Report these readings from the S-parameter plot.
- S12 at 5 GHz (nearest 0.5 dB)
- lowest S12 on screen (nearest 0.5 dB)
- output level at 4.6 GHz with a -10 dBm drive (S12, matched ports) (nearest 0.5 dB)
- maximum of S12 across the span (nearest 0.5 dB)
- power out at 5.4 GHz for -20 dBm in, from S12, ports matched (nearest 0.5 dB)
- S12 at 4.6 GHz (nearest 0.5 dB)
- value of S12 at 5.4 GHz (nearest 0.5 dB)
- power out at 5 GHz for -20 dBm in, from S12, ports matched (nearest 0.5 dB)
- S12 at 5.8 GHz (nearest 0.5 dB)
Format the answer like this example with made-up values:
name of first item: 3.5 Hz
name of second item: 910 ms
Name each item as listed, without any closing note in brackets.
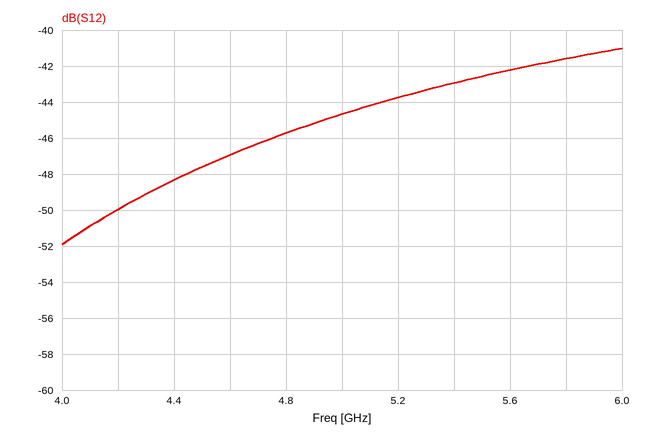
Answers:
S12 at 5 GHz: -44.5 dB
lowest S12 on screen: -52.0 dB
output level at 4.6 GHz with a -10 dBm drive (S12, matched ports): -57.0 dBm
maximum of S12 across the span: -41.0 dB
power out at 5.4 GHz for -20 dBm in, from S12, ports matched: -63.0 dBm
S12 at 4.6 GHz: -47.0 dB
value of S12 at 5.4 GHz: -43.0 dB
power out at 5 GHz for -20 dBm in, from S12, ports matched: -64.5 dBm
S12 at 5.8 GHz: -41.5 dB
